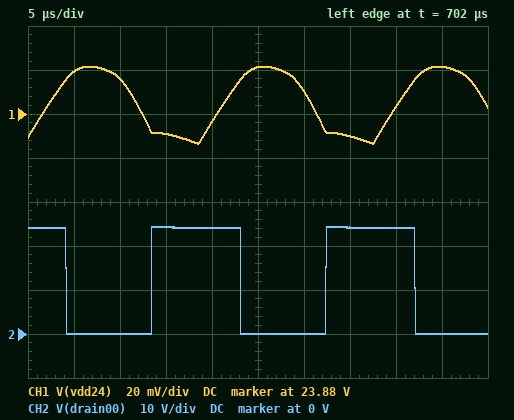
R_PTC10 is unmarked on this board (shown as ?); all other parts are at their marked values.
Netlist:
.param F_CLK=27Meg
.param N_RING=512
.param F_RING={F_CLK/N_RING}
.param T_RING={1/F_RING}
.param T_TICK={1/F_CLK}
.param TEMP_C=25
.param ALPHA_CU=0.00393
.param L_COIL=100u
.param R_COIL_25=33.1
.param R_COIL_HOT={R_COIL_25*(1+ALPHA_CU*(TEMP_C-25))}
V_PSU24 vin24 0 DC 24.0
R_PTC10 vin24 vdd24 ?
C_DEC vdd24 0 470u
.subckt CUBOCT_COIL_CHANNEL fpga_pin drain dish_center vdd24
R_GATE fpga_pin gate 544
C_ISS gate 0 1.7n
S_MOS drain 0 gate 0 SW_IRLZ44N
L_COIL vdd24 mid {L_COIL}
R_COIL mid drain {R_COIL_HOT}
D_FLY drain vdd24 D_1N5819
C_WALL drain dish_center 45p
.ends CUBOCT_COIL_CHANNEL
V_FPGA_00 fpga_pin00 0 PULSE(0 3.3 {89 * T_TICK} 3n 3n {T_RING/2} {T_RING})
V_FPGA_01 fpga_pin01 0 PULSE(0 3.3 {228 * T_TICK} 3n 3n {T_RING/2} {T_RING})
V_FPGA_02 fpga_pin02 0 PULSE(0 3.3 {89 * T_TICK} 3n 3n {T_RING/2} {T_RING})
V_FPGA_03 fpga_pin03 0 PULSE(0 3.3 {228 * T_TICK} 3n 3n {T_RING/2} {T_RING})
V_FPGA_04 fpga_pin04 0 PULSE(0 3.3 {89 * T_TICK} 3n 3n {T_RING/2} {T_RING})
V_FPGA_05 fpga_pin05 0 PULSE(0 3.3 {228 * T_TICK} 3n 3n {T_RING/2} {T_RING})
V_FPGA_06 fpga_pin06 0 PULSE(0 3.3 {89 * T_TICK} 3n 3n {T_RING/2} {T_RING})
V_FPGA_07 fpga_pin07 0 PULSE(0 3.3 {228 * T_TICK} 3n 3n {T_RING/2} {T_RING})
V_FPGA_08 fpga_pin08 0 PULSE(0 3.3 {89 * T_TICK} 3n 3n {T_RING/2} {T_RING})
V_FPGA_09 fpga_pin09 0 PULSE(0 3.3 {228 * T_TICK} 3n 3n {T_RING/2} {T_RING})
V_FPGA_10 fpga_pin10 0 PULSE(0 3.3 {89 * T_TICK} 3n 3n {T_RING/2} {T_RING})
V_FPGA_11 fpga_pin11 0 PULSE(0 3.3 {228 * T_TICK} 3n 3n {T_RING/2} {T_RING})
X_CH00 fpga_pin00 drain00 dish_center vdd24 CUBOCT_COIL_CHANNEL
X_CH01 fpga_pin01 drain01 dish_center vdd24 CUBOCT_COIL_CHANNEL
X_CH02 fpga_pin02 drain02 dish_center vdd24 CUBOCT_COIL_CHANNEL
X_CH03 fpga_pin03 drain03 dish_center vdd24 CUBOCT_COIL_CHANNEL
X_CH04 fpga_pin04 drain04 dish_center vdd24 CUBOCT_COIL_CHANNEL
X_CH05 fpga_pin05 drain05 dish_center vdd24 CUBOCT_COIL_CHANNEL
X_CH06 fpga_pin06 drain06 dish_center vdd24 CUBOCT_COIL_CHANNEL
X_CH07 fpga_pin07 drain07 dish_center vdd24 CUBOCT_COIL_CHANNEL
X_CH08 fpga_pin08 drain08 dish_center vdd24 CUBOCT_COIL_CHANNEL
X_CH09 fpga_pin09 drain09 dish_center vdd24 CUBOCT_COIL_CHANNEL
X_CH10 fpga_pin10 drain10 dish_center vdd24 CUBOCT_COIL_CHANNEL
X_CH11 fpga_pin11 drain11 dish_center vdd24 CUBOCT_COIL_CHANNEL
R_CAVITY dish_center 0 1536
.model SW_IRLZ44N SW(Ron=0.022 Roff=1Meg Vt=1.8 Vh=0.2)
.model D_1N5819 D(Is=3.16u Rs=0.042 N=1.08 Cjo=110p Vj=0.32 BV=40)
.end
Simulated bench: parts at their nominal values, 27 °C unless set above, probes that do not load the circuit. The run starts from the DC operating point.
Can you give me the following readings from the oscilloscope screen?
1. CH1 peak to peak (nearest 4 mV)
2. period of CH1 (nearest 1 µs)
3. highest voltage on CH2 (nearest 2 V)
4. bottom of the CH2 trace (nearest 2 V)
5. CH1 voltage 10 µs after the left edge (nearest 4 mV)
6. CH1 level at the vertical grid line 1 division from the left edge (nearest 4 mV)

36 mV
19 µs
24 V
0 V
23.896 V
23.900 V
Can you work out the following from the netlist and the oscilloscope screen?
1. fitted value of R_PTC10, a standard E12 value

0.039 Ω
